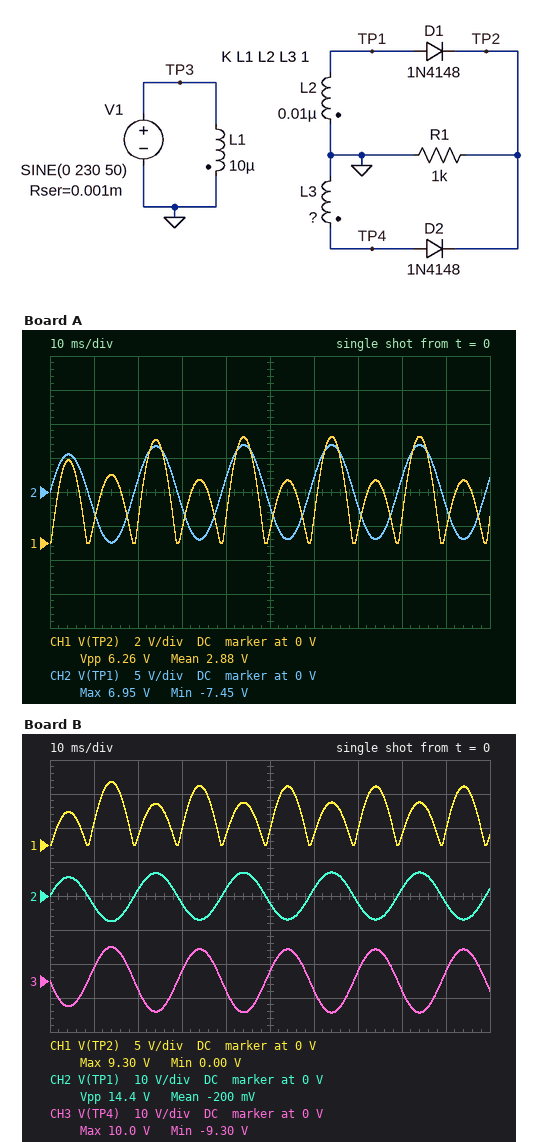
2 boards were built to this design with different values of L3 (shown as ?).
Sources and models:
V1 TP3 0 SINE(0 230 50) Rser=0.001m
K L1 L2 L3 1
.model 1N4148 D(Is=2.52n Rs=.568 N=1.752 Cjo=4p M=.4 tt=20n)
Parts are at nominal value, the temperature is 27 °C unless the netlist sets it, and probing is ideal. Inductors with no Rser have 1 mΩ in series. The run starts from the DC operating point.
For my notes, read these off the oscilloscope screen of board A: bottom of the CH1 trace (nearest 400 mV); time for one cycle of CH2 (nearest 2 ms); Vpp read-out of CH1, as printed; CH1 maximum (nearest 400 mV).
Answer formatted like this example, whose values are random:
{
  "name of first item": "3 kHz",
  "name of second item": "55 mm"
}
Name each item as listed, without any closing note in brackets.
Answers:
{
  "bottom of the CH1 trace": "0 V",
  "time for one cycle of CH2": "20 ms",
  "Vpp read-out of CH1, as printed": "6.26 V",
  "CH1 maximum": "6.4 V"
}
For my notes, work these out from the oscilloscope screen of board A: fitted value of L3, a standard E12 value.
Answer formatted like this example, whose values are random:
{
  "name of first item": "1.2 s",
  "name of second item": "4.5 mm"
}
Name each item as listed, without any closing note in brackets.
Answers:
{
  "fitted value of L3, a standard E12 value": "3.9 nH"
}
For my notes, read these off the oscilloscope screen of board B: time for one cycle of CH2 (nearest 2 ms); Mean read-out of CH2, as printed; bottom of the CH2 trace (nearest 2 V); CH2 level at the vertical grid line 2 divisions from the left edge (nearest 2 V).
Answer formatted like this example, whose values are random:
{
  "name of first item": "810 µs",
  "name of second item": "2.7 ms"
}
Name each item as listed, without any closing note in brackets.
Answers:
{
  "time for one cycle of CH2": "20 ms",
  "Mean read-out of CH2, as printed": "-200 mV",
  "bottom of the CH2 trace": "-8 V",
  "CH2 level at the vertical grid line 2 divisions from the left edge": "2 V"
}
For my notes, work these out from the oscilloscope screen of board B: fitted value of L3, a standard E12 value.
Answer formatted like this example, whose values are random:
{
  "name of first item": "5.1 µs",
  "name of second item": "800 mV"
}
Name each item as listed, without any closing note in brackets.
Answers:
{
  "fitted value of L3, a standard E12 value": "18 nH"
}
